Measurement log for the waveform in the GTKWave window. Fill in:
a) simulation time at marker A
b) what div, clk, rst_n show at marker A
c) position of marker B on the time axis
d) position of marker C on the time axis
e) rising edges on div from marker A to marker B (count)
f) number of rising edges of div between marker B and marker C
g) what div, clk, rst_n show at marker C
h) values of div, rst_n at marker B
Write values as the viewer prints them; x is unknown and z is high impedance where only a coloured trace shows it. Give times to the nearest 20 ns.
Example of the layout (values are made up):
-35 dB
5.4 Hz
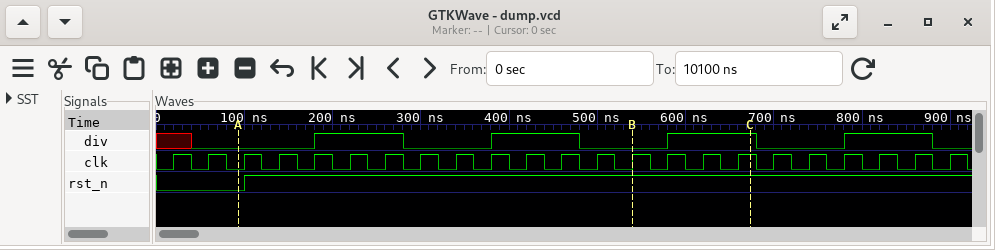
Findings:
100 ns
div=0, clk=0, rst_n=0
540 ns
680 ns
2
1
div=1, clk=1, rst_n=1
div=0, rst_n=1
